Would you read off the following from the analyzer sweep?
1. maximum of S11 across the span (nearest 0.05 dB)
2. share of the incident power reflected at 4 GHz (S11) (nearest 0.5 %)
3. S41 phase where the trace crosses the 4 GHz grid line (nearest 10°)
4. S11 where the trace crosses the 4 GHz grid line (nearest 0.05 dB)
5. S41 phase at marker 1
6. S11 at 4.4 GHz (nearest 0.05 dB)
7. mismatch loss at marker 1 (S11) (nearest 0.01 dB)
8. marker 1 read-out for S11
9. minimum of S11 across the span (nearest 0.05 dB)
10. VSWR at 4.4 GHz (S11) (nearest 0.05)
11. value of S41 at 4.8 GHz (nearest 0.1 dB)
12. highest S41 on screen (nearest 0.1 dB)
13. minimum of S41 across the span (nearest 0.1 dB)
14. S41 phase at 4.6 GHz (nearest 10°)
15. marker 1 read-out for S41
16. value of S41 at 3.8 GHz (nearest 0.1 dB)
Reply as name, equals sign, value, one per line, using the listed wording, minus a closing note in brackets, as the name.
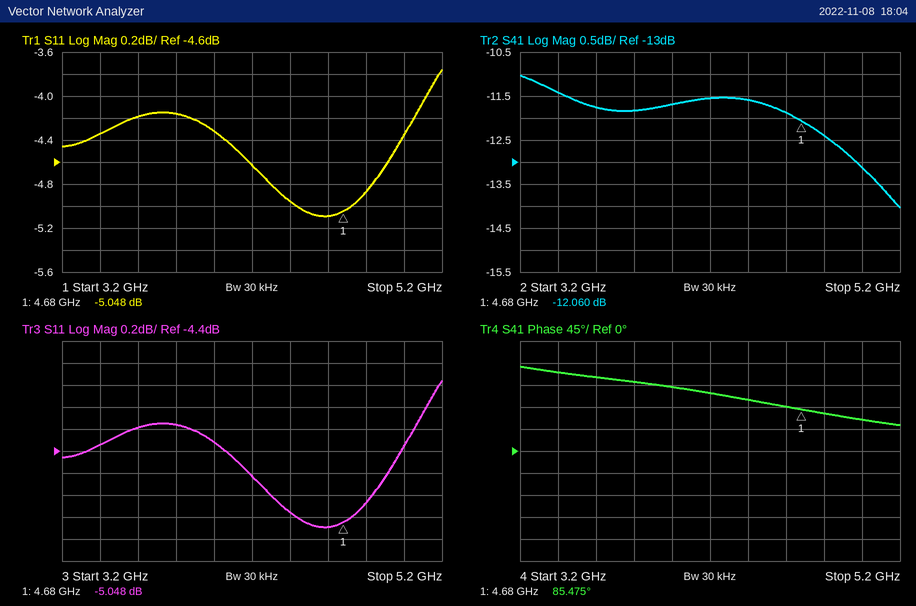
maximum of S11 across the span = -3.75 dB
share of the incident power reflected at 4 GHz (S11) = 37.0 %
S41 phase where the trace crosses the 4 GHz grid line = 130°
S11 where the trace crosses the 4 GHz grid line = -4.30 dB
S41 phase at marker 1 = 85.475°
S11 at 4.4 GHz = -4.95 dB
mismatch loss at marker 1 (S11) = 1.63 dB
marker 1 read-out for S11 = -5.048 dB
minimum of S11 across the span = -5.10 dB
VSWR at 4.4 GHz (S11) = 3.60
value of S41 at 4.8 GHz = -12.4 dB
highest S41 on screen = -11.0 dB
minimum of S41 across the span = -14.0 dB
S41 phase at 4.6 GHz = 90°
marker 1 read-out for S41 = -12.060 dB
value of S41 at 3.8 GHz = -11.8 dB
